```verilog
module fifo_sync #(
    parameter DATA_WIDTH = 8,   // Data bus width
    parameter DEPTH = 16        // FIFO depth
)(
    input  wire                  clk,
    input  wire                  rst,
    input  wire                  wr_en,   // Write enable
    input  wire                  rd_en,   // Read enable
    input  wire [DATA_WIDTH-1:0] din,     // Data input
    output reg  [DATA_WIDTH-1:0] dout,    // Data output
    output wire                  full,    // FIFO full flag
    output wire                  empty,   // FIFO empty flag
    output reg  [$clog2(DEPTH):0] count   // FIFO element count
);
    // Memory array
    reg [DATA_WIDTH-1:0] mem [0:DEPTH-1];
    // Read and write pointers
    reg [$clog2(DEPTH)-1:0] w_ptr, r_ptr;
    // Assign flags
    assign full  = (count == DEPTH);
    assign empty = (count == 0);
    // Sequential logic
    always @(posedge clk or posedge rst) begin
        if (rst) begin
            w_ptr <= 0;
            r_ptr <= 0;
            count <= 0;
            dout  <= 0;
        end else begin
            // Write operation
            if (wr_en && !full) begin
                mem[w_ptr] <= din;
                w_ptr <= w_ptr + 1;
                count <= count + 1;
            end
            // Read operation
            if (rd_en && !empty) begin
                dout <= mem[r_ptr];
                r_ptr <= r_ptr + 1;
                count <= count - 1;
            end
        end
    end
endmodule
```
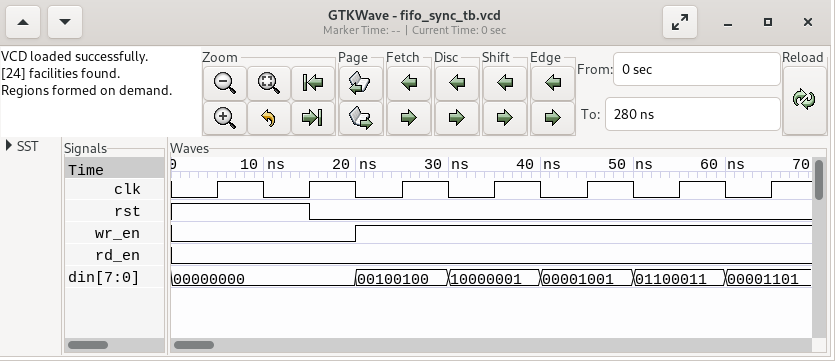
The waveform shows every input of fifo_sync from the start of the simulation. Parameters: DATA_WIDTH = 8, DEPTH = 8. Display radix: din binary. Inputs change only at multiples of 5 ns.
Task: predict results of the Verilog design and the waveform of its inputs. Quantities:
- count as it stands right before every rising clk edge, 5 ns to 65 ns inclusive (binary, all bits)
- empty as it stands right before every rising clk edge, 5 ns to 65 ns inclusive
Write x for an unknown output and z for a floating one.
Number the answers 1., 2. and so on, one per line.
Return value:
1. 0000, 0000, 0000, 0001, 0010, 0011, 0100
2. 1 1 1 0 0 0 0
